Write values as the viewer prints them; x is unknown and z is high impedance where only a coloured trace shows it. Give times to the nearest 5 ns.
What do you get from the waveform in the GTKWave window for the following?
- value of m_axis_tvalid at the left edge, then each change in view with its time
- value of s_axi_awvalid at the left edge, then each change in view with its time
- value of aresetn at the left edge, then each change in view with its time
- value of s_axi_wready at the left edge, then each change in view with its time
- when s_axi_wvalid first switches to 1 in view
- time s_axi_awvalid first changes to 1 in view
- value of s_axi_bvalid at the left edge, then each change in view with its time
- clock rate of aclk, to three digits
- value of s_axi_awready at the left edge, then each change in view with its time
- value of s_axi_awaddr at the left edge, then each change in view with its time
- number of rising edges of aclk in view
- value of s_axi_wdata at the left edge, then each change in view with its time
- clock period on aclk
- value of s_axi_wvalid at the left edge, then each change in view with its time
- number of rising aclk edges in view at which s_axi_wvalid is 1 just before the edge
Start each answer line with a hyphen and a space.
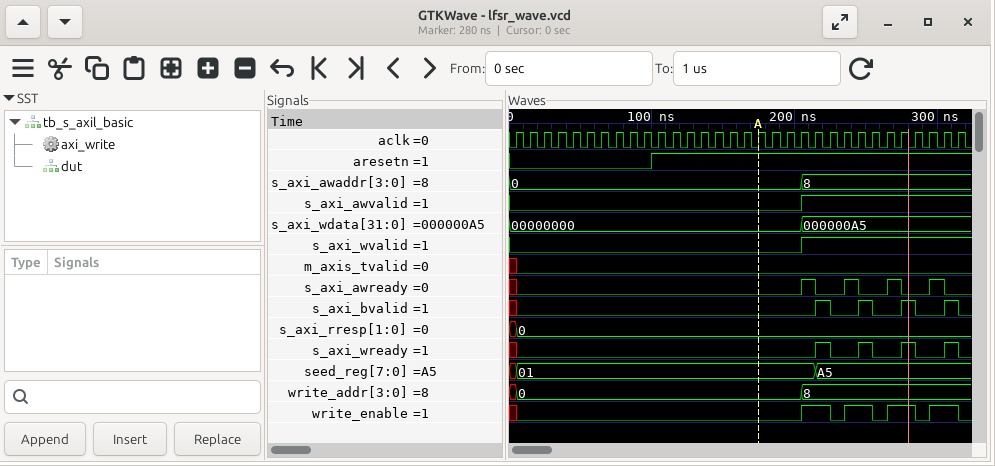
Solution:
- x, 0 at 5 ns
- 0, 1 at 205 ns
- 0, 1 at 100 ns
- x, 0 at 5 ns, 1 at 215 ns, 0 at 225 ns, 1 at 245 ns, 0 at 255 ns, 1 at 275 ns, 0 at 285 ns, 1 at 305 ns, 0 at 315 ns
- 205 ns
- 205 ns
- x, 0 at 5 ns, 1 at 215 ns, 0 at 225 ns, 1 at 245 ns, 0 at 255 ns, 1 at 275 ns, 0 at 285 ns, 1 at 305 ns, 0 at 315 ns
- 100 MHz
- x, 0 at 5 ns, 1 at 205 ns, 0 at 215 ns, 1 at 235 ns, 0 at 245 ns, 1 at 265 ns, 0 at 275 ns, 1 at 295 ns, 0 at 305 ns
- 0, 8 at 205 ns
- 32
- 00000000, 000000A5 at 205 ns
- 10 ns
- 0, 1 at 205 ns
- 11
